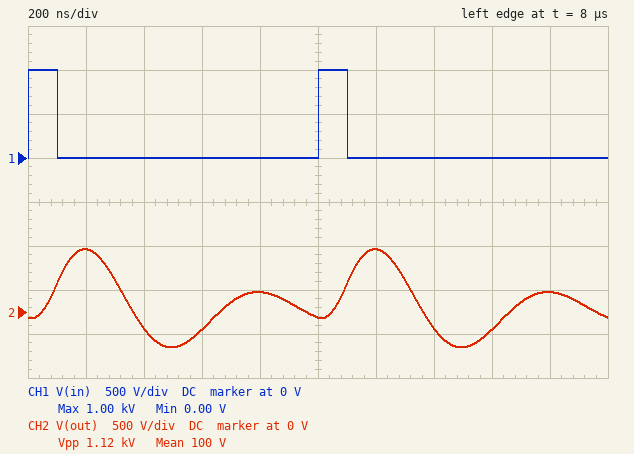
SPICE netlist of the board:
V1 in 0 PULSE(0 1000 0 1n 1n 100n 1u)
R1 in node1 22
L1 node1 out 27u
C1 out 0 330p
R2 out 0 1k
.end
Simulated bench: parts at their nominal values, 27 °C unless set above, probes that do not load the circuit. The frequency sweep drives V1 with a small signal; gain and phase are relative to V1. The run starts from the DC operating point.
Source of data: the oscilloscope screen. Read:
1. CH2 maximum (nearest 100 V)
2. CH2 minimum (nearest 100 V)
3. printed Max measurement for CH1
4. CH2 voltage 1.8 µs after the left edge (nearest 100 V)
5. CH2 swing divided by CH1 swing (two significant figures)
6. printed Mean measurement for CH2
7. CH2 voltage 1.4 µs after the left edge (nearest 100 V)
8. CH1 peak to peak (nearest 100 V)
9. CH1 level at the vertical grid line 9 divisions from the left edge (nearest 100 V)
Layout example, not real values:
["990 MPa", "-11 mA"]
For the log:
["700 V", "-400 V", "1.00 kV", "200 V", "1.1", "100 V", "-200 V", "1.0 kV", "0 V"]
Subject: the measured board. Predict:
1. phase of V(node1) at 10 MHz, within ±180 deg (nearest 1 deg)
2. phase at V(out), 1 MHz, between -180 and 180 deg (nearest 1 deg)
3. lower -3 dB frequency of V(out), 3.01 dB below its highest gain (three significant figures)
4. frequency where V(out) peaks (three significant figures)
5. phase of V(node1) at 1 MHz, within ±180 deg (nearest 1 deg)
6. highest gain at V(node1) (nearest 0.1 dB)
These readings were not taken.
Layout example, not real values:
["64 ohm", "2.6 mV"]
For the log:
["1 deg", "-18 deg", "1.30 MHz", "1.65 MHz", "-3 deg", "0 dB"]
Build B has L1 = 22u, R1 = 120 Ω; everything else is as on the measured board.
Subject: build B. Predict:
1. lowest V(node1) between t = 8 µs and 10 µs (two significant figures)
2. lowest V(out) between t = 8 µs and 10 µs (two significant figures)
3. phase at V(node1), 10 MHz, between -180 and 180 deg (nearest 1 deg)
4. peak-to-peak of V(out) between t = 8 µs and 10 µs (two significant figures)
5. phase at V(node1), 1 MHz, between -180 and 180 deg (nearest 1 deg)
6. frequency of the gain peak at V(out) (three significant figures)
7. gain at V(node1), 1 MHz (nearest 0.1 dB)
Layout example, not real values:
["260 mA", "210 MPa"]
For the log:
["-340 V", "-220 V", "5 deg", "890 V", "-14 deg", "1.73 MHz", "-2.0 dB"]
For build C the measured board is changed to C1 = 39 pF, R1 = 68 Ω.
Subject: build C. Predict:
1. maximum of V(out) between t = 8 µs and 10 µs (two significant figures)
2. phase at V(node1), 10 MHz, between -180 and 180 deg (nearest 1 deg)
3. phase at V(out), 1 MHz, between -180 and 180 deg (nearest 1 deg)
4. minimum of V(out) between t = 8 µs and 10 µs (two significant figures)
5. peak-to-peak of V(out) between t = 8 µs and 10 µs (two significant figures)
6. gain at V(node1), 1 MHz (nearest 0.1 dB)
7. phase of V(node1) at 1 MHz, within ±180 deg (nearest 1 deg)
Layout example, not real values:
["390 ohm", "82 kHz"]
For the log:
["1.1 kV", "3 deg", "-10 deg", "-240 V", "1.4 kV", "-0.6 dB", "0 deg"]
